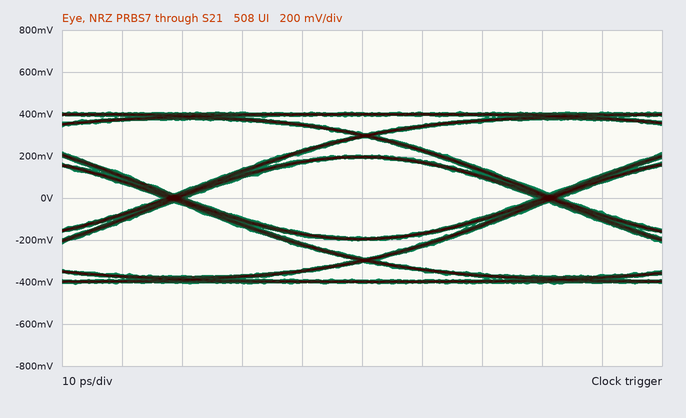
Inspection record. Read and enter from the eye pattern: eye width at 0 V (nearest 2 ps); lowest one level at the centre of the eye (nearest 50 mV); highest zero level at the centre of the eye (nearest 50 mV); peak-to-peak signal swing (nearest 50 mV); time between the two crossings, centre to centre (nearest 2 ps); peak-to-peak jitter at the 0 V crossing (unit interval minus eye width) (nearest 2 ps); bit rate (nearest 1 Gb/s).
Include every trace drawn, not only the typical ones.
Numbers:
58 ps
200 mV
-200 mV
800 mV
62 ps
4 ps
16 Gb/s
